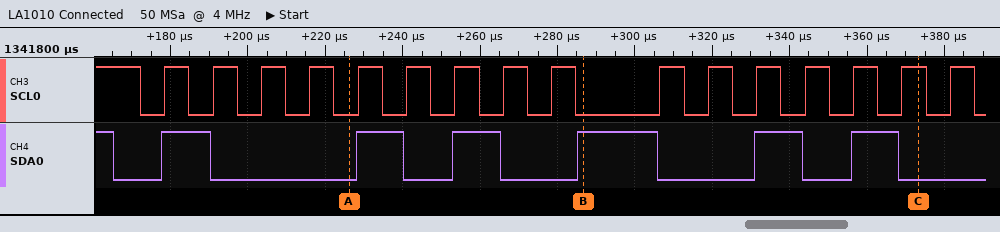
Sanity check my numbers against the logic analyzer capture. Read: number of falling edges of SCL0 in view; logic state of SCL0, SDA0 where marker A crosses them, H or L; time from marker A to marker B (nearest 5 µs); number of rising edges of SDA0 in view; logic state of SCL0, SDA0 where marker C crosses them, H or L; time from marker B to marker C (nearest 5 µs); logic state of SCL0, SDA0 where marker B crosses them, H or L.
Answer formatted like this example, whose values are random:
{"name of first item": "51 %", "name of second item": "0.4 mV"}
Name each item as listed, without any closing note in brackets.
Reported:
{"number of falling edges of SCL0 in view": "17", "logic state of SCL0, SDA0 where marker A crosses them, H or L": "SCL0=L, SDA0=L", "time from marker A to marker B": "60 µs", "number of rising edges of SDA0 in view": "6", "logic state of SCL0, SDA0 where marker C crosses them, H or L": "SCL0=H, SDA0=L", "time from marker B to marker C": "85 µs", "logic state of SCL0, SDA0 where marker B crosses them, H or L": "SCL0=L, SDA0=H"}
